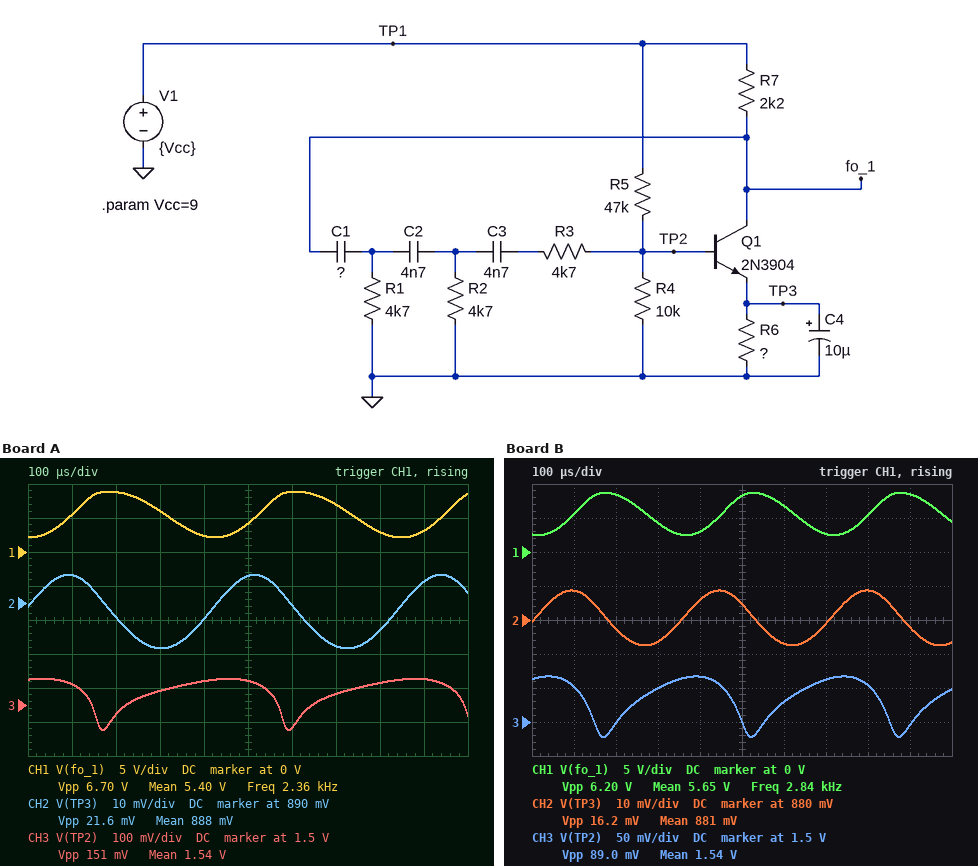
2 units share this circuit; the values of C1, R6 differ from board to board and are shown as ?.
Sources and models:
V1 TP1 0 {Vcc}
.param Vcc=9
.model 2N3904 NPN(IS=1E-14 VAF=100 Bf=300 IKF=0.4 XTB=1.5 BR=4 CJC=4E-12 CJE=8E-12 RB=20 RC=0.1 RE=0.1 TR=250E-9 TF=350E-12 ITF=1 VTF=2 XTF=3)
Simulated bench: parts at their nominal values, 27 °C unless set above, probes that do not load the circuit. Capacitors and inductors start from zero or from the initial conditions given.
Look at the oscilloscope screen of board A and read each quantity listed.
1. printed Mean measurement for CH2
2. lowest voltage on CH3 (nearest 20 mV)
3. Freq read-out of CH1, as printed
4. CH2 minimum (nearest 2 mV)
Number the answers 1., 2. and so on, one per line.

1. 888 mV
2. 1.42 V
3. 2.36 kHz
4. 876 mV
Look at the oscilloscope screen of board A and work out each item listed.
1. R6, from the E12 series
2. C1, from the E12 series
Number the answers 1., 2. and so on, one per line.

1. 560 Ω
2. 3.9 nF
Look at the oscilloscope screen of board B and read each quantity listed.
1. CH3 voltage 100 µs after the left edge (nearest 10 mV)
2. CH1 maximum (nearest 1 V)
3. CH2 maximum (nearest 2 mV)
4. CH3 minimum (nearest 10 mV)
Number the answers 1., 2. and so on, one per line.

1. 1.55 V
2. 9 V
3. 888 mV
4. 1.48 V
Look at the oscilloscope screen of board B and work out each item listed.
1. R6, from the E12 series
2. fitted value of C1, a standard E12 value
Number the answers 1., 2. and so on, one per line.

1. 560 Ω
2. 2.2 nF
